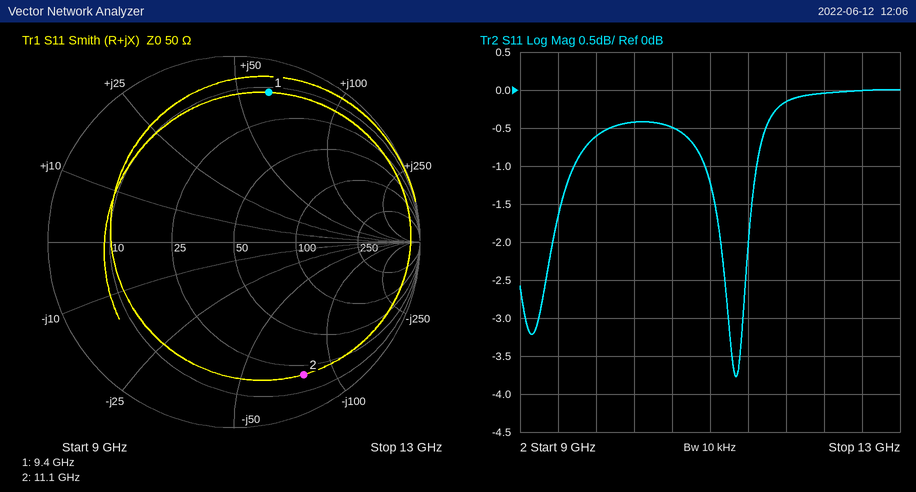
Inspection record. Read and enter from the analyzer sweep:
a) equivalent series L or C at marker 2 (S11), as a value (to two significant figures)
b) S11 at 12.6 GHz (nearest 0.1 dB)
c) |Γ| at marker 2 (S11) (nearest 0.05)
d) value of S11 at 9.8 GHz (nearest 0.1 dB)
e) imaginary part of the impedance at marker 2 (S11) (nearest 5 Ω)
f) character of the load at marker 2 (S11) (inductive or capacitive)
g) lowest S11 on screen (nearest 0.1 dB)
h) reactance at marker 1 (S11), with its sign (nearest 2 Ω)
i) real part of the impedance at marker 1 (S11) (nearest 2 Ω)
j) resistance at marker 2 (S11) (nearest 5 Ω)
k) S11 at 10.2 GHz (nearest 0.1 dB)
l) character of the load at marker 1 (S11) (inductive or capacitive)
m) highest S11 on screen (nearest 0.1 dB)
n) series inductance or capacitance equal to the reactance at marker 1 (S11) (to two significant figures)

180 fF
0.0 dB
0.80
-0.6 dB
-80 Ω
capacitive
-3.8 dB
+62 Ω
12 Ω
20 Ω
-0.4 dB
inductive
0.0 dB
1.0 nH
